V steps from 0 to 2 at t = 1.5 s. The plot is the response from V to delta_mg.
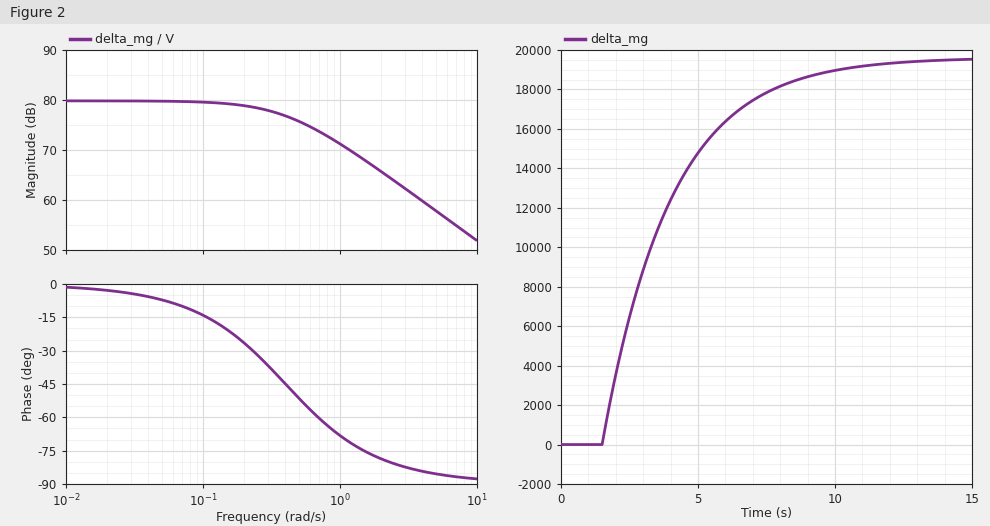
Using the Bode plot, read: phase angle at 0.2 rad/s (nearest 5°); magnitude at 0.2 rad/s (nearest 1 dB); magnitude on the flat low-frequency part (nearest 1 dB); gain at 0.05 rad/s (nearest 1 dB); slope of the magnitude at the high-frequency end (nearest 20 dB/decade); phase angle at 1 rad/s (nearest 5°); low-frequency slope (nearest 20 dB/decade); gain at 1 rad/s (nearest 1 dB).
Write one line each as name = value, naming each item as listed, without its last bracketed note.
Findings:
phase angle at 0.2 rad/s = -25°
magnitude at 0.2 rad/s = 79 dB
magnitude on the flat low-frequency part = 80 dB
gain at 0.05 rad/s = 80 dB
slope of the magnitude at the high-frequency end = -20 dB/decade
phase angle at 1 rad/s = -70°
low-frequency slope = 0 dB/decade
gain at 1 rad/s = 71 dB
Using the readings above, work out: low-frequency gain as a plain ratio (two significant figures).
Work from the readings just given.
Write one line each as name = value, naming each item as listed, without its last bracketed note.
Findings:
low-frequency gain as a plain ratio = 10000
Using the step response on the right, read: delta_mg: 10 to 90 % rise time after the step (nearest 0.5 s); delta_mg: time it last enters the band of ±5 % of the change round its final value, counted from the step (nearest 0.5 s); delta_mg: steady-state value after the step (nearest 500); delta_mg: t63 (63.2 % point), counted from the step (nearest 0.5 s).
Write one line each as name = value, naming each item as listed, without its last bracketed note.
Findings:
delta_mg: 10 to 90 % rise time after the step = 5.5 s
delta_mg: time it last enters the band of ±5 % of the change round its final value, counted from the step = 7.5 s
delta_mg: steady-state value after the step = 19500
delta_mg: t63 (63.2 % point), counted from the step = 2.5 s
